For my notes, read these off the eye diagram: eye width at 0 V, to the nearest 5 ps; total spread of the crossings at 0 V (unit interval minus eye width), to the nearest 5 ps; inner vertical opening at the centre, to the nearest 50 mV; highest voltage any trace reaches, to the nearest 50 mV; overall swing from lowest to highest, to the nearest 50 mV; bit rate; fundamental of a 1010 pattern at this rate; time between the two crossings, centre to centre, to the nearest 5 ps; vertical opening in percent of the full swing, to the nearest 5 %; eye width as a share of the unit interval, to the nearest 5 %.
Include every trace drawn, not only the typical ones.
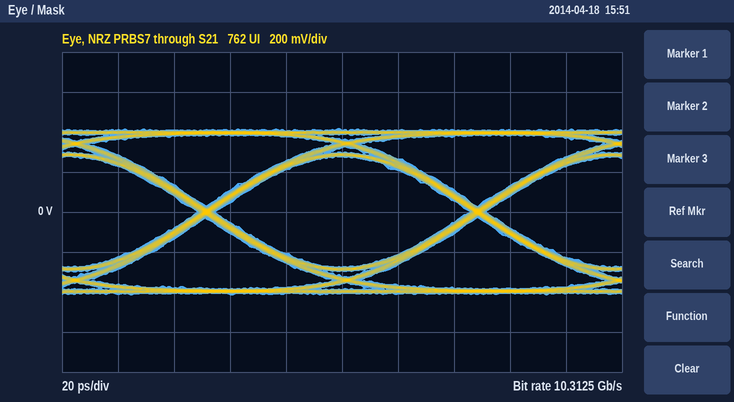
90 ps
5 ps
550 mV
400 mV
850 mV
10.3125 Gb/s
5.15625 GHz
95 ps
65 %
95 %
